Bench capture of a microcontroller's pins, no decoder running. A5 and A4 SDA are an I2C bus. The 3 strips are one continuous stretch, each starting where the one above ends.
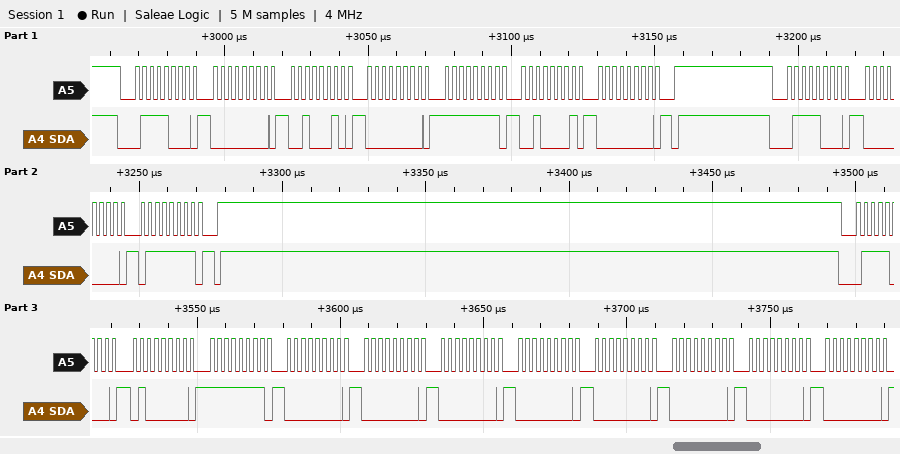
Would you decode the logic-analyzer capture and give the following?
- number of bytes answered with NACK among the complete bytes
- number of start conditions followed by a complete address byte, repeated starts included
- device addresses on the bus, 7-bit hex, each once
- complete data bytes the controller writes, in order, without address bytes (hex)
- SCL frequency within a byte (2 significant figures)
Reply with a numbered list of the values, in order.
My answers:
1. 0
2. 3
3. 0x3C
4. 00 22 00 FF 21 00 00 7F 40 FF 00 00 00 00 00 00 00 00
5. 400 kHz
